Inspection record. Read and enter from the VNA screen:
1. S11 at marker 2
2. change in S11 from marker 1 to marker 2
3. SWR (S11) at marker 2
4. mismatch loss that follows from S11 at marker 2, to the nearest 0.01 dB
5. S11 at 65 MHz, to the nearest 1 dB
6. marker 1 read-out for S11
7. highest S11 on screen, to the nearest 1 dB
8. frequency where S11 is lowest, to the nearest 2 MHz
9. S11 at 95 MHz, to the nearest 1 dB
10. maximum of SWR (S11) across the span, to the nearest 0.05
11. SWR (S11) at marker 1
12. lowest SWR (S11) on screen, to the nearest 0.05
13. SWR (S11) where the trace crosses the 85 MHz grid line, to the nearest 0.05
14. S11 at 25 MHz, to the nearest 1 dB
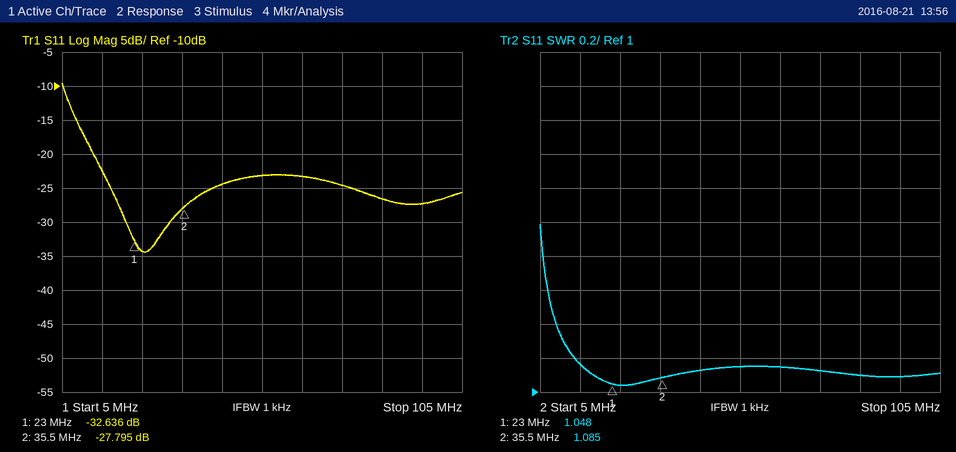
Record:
-27.795 dB
4.841 dB
1.085
0.01 dB
-23 dB
-32.636 dB
-10 dB
26 MHz
-27 dB
2.00
1.048
1.05
1.10
-34 dB
